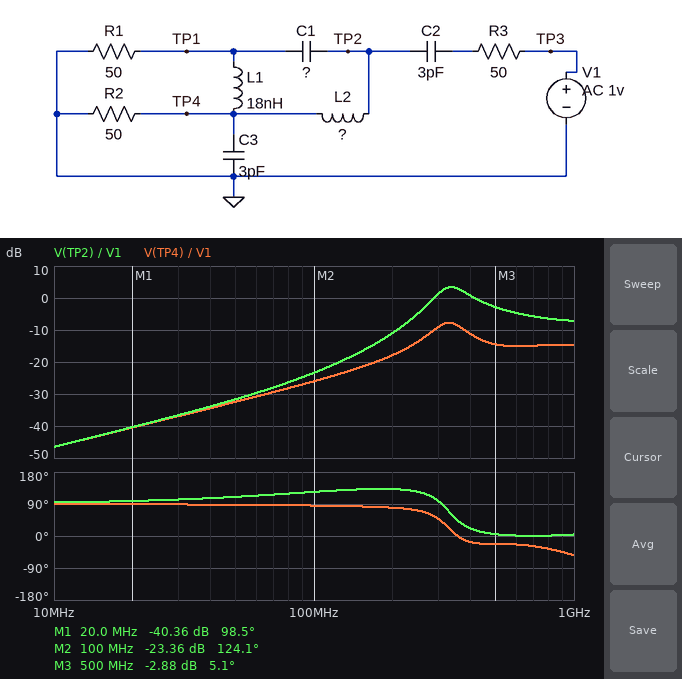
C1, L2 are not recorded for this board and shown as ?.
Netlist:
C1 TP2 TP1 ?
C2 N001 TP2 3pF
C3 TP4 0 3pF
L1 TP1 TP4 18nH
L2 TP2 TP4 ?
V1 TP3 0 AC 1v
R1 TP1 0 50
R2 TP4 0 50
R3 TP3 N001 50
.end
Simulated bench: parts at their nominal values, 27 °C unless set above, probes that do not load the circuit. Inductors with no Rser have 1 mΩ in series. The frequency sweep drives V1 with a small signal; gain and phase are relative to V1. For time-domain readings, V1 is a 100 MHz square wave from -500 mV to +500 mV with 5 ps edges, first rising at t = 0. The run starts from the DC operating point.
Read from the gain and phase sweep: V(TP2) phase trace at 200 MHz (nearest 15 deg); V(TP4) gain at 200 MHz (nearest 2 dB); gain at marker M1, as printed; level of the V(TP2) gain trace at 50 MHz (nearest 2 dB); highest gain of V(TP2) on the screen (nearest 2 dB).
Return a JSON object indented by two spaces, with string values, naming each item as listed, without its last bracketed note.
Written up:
{
  "V(TP2) phase trace at 200 MHz": "135 deg",
  "V(TP4) gain at 200 MHz": "-18 dB",
  "gain at marker M1, as printed": "-40.36 dB",
  "level of the V(TP2) gain trace at 50 MHz": "-32 dB",
  "highest gain of V(TP2) on the screen": "4 dB"
}
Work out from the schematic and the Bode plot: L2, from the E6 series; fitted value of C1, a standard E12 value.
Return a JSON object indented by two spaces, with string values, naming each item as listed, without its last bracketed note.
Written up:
{
  "L2, from the E6 series": "33 nH",
  "fitted value of C1, a standard E12 value": "2.7 pF"
}
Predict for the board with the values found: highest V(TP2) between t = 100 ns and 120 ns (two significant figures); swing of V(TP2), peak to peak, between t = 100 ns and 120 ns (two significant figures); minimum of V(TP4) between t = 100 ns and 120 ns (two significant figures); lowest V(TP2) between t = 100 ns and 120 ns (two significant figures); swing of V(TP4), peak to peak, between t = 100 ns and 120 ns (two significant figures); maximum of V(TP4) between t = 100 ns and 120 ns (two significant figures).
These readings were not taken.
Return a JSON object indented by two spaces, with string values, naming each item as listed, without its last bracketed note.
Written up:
{
  "highest V(TP2) between t = 100 ns and 120 ns": "570 mV",
  "swing of V(TP2), peak to peak, between t = 100 ns and 120 ns": "1.1 V",
  "minimum of V(TP4) between t = 100 ns and 120 ns": "-180 mV",
  "lowest V(TP2) between t = 100 ns and 120 ns": "-570 mV",
  "swing of V(TP4), peak to peak, between t = 100 ns and 120 ns": "350 mV",
  "maximum of V(TP4) between t = 100 ns and 120 ns": "180 mV"
}
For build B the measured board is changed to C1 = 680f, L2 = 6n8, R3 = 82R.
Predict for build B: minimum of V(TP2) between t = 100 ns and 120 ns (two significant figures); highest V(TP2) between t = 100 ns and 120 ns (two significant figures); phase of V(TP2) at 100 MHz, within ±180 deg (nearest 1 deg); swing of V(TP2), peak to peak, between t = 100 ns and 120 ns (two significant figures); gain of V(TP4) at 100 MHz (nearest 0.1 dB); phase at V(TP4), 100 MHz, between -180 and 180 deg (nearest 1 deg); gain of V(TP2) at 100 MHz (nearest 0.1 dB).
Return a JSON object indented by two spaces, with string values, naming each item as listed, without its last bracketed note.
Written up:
{
  "minimum of V(TP2) between t = 100 ns and 120 ns": "-450 mV",
  "highest V(TP2) between t = 100 ns and 120 ns": "450 mV",
  "phase of V(TP2) at 100 MHz, within ±180 deg": "91 deg",
  "swing of V(TP2), peak to peak, between t = 100 ns and 120 ns": "890 mV",
  "gain of V(TP4) at 100 MHz": "-26.4 dB",
  "phase at V(TP4), 100 MHz, between -180 and 180 deg": "82 deg",
  "gain of V(TP2) at 100 MHz": "-26.2 dB"
}
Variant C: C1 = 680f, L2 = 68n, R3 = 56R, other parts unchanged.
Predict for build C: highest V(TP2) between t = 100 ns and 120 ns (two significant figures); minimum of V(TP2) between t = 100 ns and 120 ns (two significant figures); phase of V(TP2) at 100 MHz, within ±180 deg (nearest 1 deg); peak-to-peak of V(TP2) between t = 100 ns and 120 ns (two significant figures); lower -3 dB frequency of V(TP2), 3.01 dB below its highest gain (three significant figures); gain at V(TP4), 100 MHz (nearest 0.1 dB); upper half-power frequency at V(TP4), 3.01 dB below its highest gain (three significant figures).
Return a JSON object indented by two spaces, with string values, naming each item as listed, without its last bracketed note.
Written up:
{
  "highest V(TP2) between t = 100 ns and 120 ns": "810 mV",
  "minimum of V(TP2) between t = 100 ns and 120 ns": "-810 mV",
  "phase of V(TP2) at 100 MHz, within ±180 deg": "141 deg",
  "peak-to-peak of V(TP2) between t = 100 ns and 120 ns": "1.6 V",
  "lower -3 dB frequency of V(TP2), 3.01 dB below its highest gain": "270 MHz",
  "gain at V(TP4), 100 MHz": "-25.7 dB",
  "upper half-power frequency at V(TP4), 3.01 dB below its highest gain": "389 MHz"
}
